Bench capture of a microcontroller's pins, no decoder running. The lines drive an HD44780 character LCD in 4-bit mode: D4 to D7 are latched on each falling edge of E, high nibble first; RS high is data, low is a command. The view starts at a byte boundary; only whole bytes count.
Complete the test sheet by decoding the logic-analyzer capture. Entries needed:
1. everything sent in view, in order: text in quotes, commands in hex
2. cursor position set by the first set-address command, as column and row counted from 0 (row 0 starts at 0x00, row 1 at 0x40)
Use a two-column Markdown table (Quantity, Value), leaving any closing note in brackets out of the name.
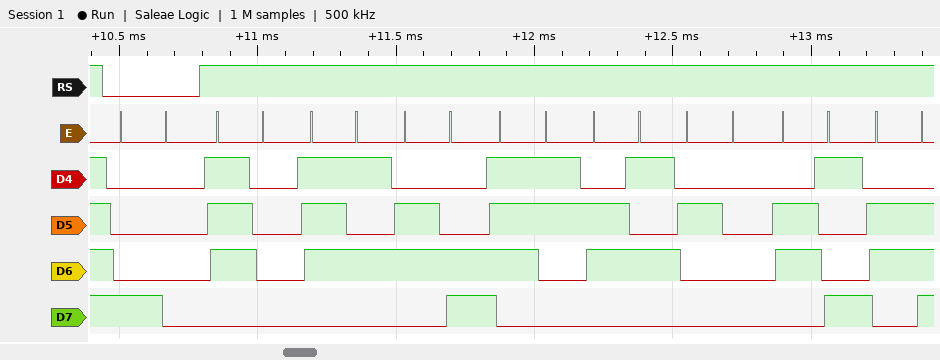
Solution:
| Quantity | Value |
|---|---|
| everything sent in view, in order: text in quotes, commands in hex | 0x80 "pulse in" |
| cursor position set by the first set-address command, as column and row counted from 0 | column 0, row 0 |
